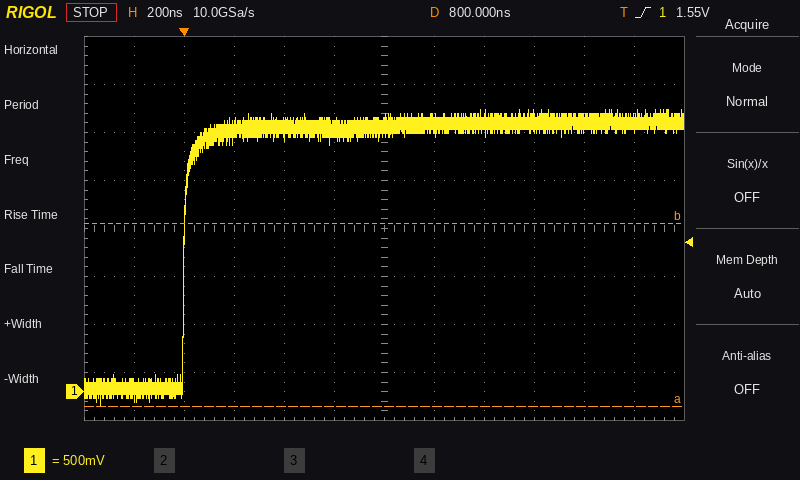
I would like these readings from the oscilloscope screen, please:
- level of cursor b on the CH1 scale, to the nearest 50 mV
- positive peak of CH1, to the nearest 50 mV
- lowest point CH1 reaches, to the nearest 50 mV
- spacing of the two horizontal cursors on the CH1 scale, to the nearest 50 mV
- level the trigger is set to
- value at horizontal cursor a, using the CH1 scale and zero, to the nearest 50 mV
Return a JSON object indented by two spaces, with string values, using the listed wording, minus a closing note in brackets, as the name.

{
  "level of cursor b on the CH1 scale, to the nearest 50 mV": "1.75 V",
  "positive peak of CH1, to the nearest 50 mV": "2.95 V",
  "lowest point CH1 reaches, to the nearest 50 mV": "-150 mV",
  "spacing of the two horizontal cursors on the CH1 scale, to the nearest 50 mV": "1.90 V",
  "level the trigger is set to": "1.55 V",
  "value at horizontal cursor a, using the CH1 scale and zero, to the nearest 50 mV": "-150 mV"
}
